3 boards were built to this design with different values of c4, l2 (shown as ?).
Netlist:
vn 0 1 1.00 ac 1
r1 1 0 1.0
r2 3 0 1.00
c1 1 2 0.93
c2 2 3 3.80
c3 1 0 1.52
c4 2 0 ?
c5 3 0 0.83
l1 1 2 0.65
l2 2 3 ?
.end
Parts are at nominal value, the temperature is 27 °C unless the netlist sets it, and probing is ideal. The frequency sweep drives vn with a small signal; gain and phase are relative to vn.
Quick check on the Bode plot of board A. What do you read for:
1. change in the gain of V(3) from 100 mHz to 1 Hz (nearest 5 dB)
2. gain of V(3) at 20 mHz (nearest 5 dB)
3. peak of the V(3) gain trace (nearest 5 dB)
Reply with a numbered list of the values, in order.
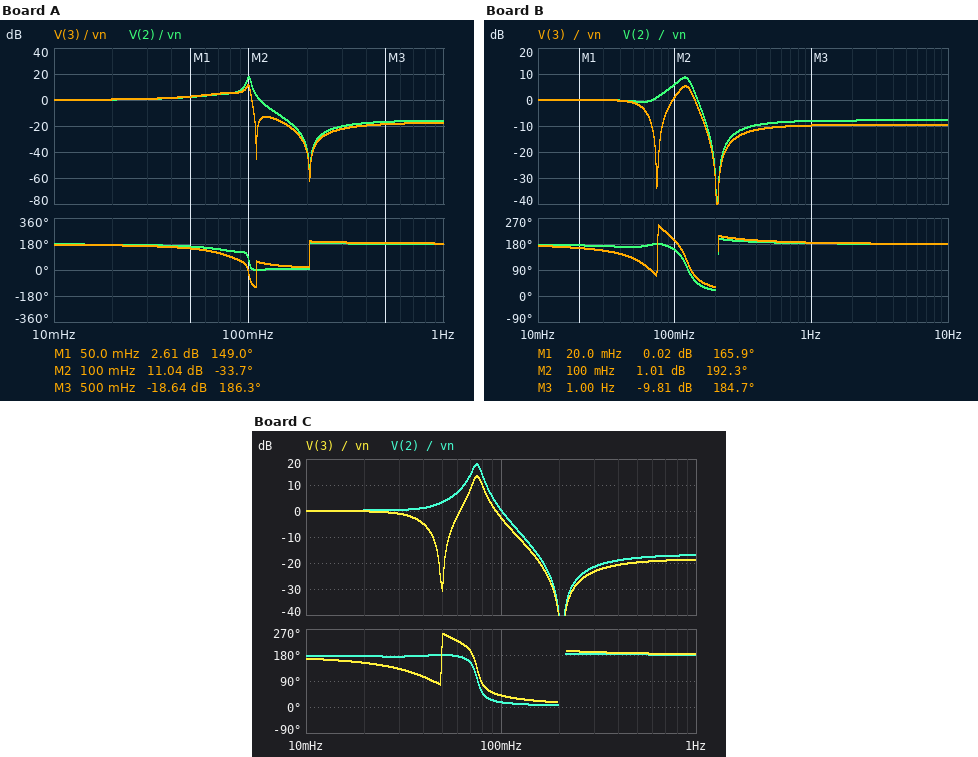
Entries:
1. -30 dB
2. 0 dB
3. 10 dB
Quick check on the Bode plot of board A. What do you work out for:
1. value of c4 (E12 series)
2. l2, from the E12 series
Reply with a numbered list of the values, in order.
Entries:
1. 3.9 F
2. 560 mH
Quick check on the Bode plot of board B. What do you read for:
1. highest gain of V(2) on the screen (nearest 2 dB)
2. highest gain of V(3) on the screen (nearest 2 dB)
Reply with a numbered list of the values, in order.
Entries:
1. 8 dB
2. 6 dB
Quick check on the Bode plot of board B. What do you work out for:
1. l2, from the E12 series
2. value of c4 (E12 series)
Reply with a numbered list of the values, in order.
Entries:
1. 1.2 H
2. 680 mF
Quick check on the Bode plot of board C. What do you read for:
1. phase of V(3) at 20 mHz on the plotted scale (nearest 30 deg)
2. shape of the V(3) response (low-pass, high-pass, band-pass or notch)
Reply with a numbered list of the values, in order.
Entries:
1. 150 deg
2. band-pass
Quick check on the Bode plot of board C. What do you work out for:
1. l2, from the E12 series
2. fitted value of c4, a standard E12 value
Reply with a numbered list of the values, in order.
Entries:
1. 2.7 H
2. 4.7 F
